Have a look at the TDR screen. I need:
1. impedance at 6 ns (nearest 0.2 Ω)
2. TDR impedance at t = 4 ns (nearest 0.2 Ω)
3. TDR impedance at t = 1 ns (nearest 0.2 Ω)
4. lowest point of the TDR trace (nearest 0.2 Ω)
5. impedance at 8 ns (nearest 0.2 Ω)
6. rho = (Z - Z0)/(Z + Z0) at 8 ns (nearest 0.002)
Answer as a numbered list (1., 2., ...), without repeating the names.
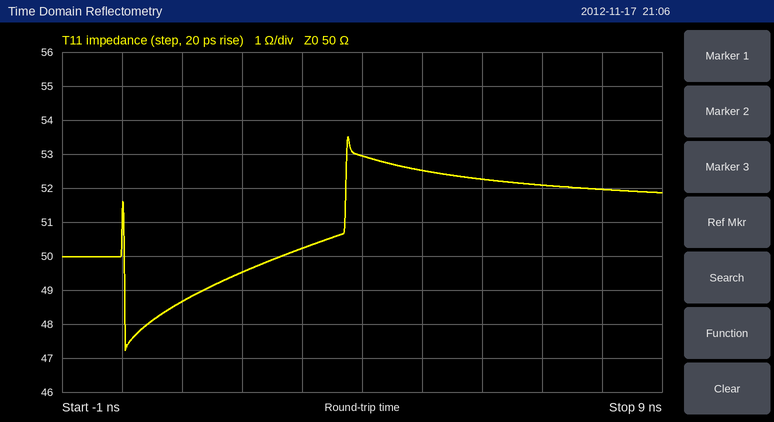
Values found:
1. 52.2 Ω
2. 53.0 Ω
3. 48.6 Ω
4. 47.2 Ω
5. 52.0 Ω
6. +0.020
